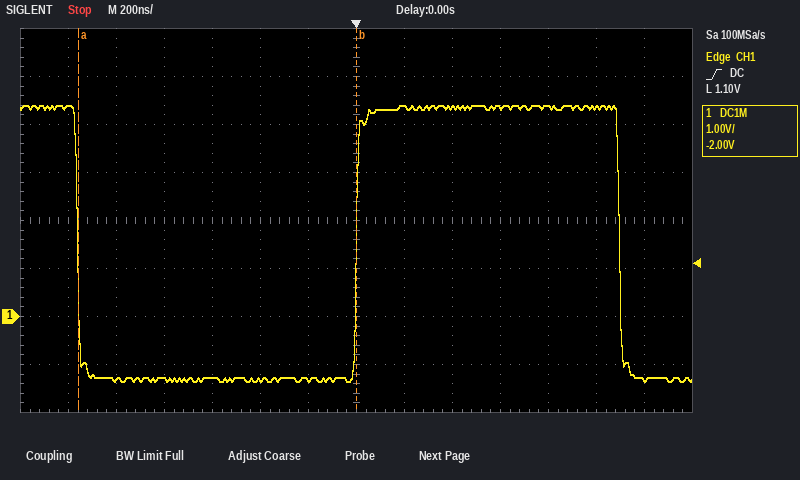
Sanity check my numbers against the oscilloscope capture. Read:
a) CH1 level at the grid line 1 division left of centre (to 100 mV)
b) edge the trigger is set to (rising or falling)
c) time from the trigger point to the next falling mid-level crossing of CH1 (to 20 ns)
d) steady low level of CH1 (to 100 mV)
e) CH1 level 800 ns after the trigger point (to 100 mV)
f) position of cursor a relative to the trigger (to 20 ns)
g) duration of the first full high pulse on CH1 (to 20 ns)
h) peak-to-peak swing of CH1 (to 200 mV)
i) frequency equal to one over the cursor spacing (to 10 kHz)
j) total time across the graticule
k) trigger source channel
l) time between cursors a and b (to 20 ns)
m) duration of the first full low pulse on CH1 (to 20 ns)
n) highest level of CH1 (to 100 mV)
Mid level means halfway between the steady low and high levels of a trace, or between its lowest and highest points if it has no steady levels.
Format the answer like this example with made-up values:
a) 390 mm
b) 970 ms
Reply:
a) -1.3 V
b) rising
c) 1.10 µs
d) -1.3 V
e) 4.4 V
f) -1.16 µs
g) 1.10 µs
h) 5.8 V
i) 860 kHz
j) 2.8 µs
k) CH1
l) 1.16 µs
m) 1.16 µs
n) 4.4 V
